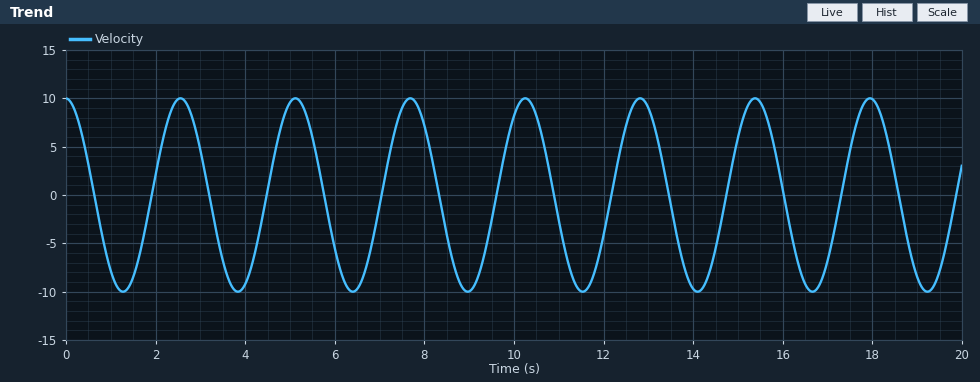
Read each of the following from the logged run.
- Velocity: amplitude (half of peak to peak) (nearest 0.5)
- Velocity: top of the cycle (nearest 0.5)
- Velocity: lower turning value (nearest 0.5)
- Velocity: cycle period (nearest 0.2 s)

10.0
10.0
-10.0
2.6 s
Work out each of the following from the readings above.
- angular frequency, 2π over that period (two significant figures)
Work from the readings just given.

2.4 rad/s
